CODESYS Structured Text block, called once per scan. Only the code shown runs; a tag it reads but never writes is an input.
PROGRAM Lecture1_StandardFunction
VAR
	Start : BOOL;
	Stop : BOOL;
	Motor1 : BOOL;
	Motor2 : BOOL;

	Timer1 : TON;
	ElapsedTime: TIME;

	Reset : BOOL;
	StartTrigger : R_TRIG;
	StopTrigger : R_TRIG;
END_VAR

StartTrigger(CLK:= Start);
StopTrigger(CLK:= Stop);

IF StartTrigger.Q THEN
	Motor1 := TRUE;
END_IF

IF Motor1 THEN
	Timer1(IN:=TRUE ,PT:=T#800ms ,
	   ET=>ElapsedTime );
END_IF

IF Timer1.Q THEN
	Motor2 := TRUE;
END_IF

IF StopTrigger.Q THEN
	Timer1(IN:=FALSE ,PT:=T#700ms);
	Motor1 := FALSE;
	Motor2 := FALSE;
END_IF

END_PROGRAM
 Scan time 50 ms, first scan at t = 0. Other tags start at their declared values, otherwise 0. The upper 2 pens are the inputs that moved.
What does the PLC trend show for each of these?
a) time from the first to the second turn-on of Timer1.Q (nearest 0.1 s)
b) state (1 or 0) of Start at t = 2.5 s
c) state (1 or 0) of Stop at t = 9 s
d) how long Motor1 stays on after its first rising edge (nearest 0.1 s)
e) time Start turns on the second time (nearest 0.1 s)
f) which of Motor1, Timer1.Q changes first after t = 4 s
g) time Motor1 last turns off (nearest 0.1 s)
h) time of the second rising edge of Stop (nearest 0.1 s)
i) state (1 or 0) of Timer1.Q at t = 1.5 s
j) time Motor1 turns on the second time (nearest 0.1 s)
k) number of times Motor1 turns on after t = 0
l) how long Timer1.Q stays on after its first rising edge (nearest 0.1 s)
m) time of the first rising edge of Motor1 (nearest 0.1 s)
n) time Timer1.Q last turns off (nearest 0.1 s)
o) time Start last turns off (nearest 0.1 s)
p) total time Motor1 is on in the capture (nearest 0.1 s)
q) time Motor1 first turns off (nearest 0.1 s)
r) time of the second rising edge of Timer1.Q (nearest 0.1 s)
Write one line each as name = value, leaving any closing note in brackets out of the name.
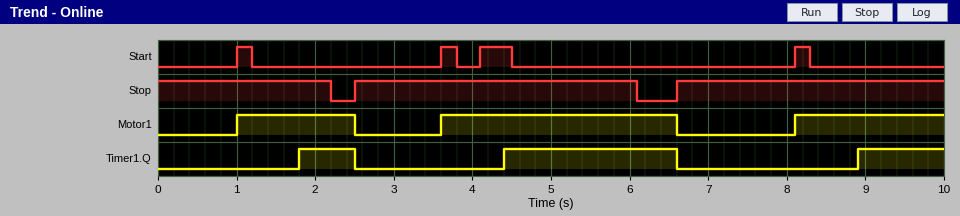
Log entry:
time from the first to the second turn-on of Timer1.Q = 2.6 s
state (1 or 0) of Start at t = 2.5 s = 0
state (1 or 0) of Stop at t = 9 s = 1
how long Motor1 stays on after its first rising edge = 1.5 s
time Start turns on the second time = 3.6 s
which of Motor1, Timer1.Q changes first after t = 4 s = Timer1.Q
time Motor1 last turns off = 6.6 s
time of the second rising edge of Stop = 6.6 s
state (1 or 0) of Timer1.Q at t = 1.5 s = 0
time Motor1 turns on the second time = 3.6 s
number of times Motor1 turns on after t = 0 = 3
how long Timer1.Q stays on after its first rising edge = 0.7 s
time of the first rising edge of Motor1 = 1.0 s
time Timer1.Q last turns off = 6.6 s
time Start last turns off = 8.3 s
total time Motor1 is on in the capture = 6.4 s
time Motor1 first turns off = 2.5 s
time of the second rising edge of Timer1.Q = 4.4 s
